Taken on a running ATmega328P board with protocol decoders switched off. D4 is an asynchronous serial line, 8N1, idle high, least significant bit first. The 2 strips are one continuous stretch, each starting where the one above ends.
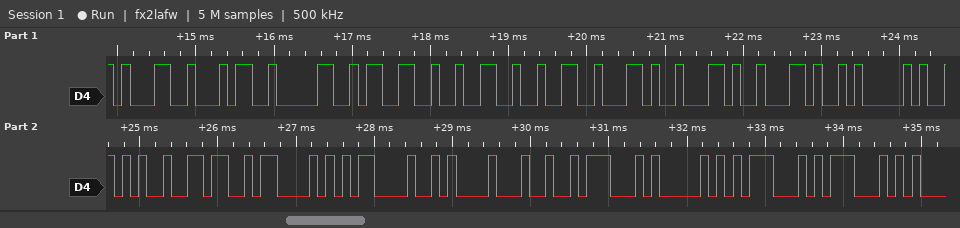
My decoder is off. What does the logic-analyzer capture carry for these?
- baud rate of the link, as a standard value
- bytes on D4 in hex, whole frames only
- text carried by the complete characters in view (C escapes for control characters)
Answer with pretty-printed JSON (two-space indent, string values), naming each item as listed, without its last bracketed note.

{
  "baud rate of the link, as a standard value": "9600 baud",
  "bytes on D4 in hex, whole frames only": "31 34 30 33 32 32 2C 2C 2C 41 2A 36 43 0D 0A 24 47 50 47 47",
  "text carried by the complete characters in view": "\"140322,,,A*6C\\r\\n$GPGG\""
}
